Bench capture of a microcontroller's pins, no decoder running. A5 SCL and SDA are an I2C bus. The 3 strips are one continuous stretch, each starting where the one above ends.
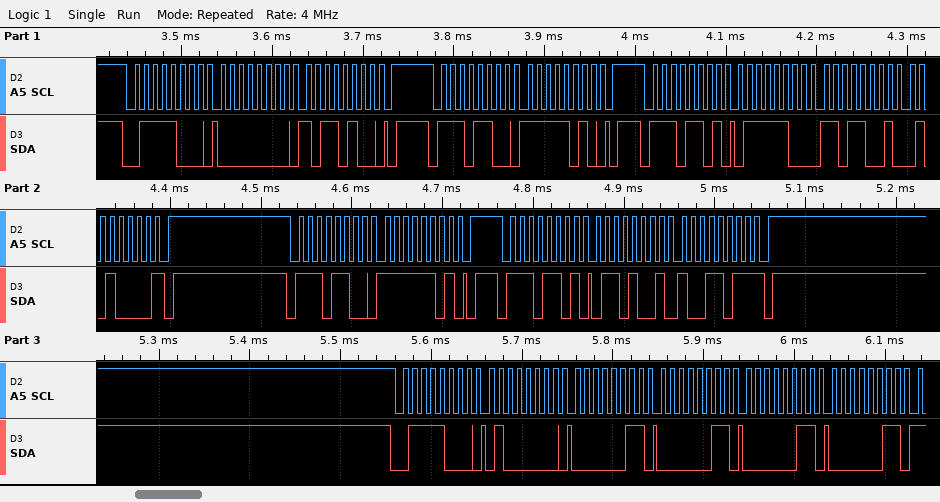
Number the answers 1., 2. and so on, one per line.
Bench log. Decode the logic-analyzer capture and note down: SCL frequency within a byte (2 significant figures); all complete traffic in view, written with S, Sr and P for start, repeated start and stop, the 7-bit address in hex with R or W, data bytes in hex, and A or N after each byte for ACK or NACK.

1. 100 kHz
2. S 3CW A 00 A B4 A P S 76W A FA A P S 76R A 7C A D9 A 50 N P S 76W A FD A P S 76R A 69 A 9B N P S 3CW A 40 A 03 A 03 A 03 A 03 A
